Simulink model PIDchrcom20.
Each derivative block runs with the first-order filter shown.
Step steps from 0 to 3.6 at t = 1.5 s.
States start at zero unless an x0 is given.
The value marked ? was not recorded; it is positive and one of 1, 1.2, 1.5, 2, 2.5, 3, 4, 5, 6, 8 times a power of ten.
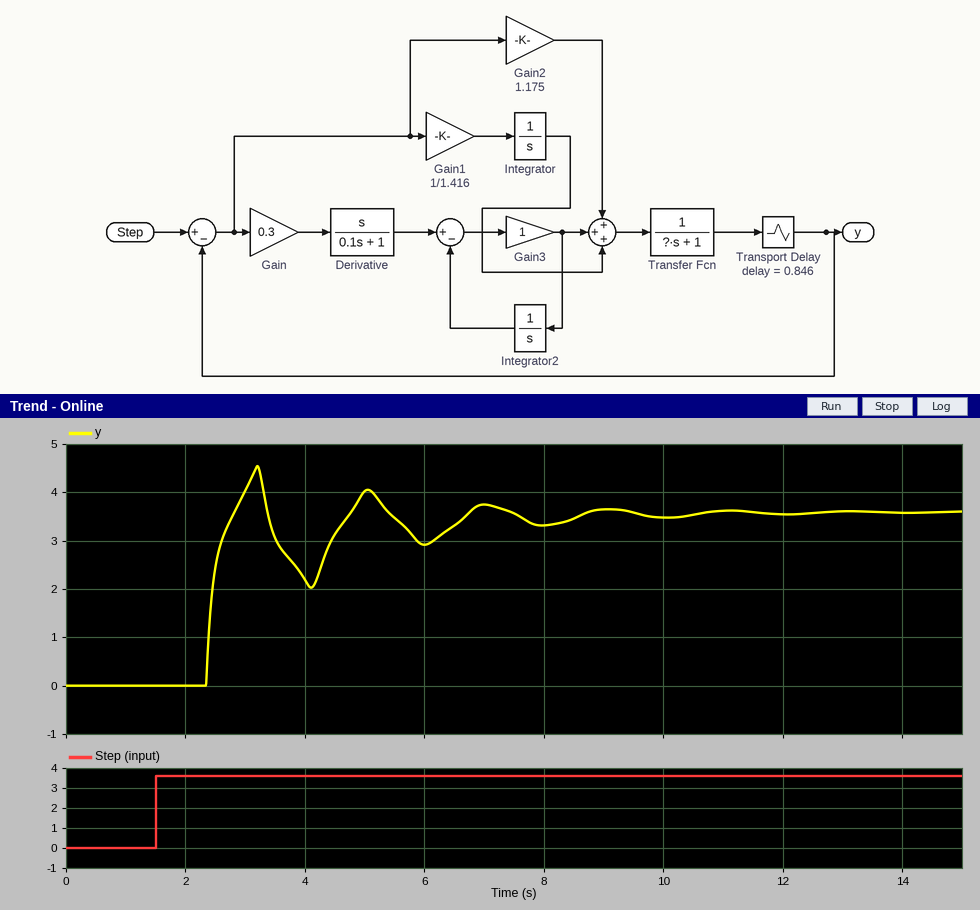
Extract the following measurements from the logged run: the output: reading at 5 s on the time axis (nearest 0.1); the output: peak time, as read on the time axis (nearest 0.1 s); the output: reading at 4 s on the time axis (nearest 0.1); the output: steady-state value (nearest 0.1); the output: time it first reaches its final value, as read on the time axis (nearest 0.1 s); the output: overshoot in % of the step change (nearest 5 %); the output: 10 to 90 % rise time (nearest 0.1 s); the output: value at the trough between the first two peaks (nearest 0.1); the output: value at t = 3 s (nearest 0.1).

4.0
3.2 s
2.2
3.6
2.8 s
25 %
0.3 s
2.0
4.0
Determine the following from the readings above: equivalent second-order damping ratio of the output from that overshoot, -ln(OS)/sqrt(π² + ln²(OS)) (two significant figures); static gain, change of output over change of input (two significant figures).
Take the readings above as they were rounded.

0.40
1.0
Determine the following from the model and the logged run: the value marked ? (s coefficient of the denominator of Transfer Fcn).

0.5
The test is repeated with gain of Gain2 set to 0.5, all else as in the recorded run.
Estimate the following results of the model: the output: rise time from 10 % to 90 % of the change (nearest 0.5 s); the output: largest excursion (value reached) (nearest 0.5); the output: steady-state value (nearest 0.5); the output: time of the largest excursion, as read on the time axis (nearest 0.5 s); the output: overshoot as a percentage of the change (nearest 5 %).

2.0 s
4.0
3.5
6.0 s
10 %
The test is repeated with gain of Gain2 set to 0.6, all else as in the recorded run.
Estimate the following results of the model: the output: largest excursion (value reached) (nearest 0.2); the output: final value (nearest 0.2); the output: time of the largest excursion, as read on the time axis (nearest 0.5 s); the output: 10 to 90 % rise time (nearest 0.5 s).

3.8
3.6
5.0 s
2.0 s
